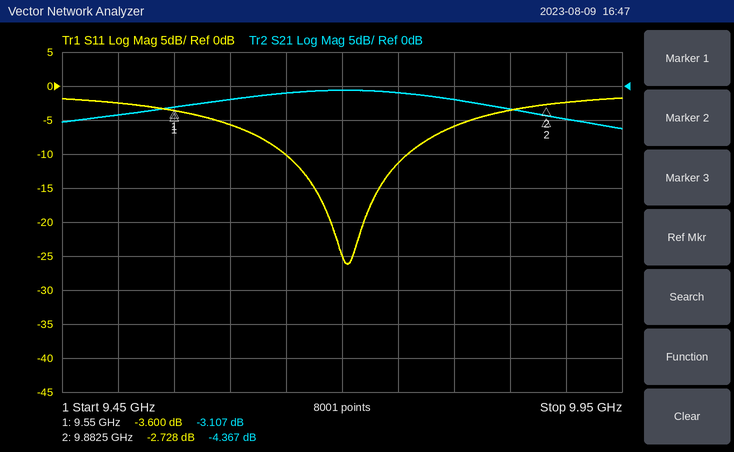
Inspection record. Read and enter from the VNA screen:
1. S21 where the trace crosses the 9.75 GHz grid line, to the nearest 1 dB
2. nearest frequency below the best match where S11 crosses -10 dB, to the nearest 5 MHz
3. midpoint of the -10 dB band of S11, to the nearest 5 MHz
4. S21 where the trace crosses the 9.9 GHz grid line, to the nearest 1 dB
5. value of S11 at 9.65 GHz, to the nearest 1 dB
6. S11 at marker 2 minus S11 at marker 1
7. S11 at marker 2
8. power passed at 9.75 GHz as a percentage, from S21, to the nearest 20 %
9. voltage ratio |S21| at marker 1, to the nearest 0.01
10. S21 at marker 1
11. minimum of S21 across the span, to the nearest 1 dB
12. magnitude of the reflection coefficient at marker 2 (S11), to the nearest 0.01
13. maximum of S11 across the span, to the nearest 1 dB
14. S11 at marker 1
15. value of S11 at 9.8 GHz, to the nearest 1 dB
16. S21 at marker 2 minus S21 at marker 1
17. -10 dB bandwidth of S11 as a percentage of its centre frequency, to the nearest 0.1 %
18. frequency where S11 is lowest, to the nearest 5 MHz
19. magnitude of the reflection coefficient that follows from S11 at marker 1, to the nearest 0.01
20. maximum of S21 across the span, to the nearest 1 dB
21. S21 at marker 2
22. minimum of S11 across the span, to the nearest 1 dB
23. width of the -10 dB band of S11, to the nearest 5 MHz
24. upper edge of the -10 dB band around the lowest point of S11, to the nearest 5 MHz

-1 dB
9.650 GHz
9.705 GHz
-5 dB
-10 dB
0.872 dB
-2.728 dB
80 %
0.70
-3.107 dB
-6 dB
0.73
-2 dB
-3.600 dB
-6 dB
-1.260 dB
1.1 %
9.705 GHz
0.66
-1 dB
-4.367 dB
-26 dB
110 MHz
9.760 GHz
